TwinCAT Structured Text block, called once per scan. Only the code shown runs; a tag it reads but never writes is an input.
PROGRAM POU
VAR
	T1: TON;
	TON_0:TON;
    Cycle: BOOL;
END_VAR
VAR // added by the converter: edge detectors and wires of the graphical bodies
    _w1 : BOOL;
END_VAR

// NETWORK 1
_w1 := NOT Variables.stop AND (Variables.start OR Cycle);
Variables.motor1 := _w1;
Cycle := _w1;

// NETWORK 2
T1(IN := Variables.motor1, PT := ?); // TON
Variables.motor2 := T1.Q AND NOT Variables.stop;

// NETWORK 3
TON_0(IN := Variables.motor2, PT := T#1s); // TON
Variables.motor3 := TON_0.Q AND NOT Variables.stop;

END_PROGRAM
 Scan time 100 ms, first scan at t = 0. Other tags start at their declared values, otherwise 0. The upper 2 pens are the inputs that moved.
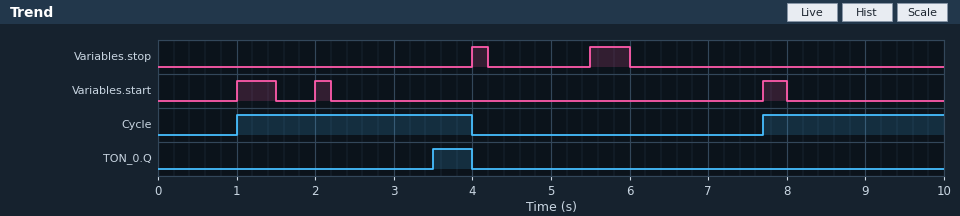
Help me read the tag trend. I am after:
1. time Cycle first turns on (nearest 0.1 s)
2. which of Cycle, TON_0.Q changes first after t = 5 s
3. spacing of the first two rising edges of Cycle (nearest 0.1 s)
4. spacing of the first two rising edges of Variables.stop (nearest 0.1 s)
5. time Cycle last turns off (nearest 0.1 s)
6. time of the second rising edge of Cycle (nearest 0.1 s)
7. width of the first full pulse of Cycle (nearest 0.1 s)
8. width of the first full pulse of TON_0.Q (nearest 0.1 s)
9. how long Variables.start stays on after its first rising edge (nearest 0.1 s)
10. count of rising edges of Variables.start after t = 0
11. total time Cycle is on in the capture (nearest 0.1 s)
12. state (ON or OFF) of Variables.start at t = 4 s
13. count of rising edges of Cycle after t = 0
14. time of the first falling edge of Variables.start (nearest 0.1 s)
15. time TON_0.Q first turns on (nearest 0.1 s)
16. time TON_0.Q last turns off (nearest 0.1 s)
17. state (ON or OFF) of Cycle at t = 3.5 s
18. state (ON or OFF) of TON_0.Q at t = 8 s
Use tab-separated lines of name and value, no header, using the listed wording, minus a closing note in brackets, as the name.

time Cycle first turns on	1.0 s
which of Cycle, TON_0.Q changes first after t = 5 s	Cycle
spacing of the first two rising edges of Cycle	6.7 s
spacing of the first two rising edges of Variables.stop	1.5 s
time Cycle last turns off	4.0 s
time of the second rising edge of Cycle	7.7 s
width of the first full pulse of Cycle	3.0 s
width of the first full pulse of TON_0.Q	0.5 s
how long Variables.start stays on after its first rising edge	0.5 s
count of rising edges of Variables.start after t = 0	3
total time Cycle is on in the capture	5.3 s
state (ON or OFF) of Variables.start at t = 4 s	OFF
count of rising edges of Cycle after t = 0	2
time of the first falling edge of Variables.start	1.5 s
time TON_0.Q first turns on	3.5 s
time TON_0.Q last turns off	4.0 s
state (ON or OFF) of Cycle at t = 3.5 s	ON
state (ON or OFF) of TON_0.Q at t = 8 s	OFF
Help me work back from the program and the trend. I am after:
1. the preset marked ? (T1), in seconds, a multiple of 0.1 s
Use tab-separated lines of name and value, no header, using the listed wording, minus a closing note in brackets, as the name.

the preset marked ? (T1), in seconds, a multiple of 0.1 s	1.5 s
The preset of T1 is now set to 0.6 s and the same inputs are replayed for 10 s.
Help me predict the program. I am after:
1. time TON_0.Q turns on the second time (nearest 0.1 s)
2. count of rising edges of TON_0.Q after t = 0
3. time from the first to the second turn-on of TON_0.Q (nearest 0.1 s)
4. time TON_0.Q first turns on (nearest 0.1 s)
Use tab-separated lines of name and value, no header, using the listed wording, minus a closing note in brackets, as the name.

time TON_0.Q turns on the second time	9.3 s
count of rising edges of TON_0.Q after t = 0	2
time from the first to the second turn-on of TON_0.Q	6.7 s
time TON_0.Q first turns on	2.6 s
